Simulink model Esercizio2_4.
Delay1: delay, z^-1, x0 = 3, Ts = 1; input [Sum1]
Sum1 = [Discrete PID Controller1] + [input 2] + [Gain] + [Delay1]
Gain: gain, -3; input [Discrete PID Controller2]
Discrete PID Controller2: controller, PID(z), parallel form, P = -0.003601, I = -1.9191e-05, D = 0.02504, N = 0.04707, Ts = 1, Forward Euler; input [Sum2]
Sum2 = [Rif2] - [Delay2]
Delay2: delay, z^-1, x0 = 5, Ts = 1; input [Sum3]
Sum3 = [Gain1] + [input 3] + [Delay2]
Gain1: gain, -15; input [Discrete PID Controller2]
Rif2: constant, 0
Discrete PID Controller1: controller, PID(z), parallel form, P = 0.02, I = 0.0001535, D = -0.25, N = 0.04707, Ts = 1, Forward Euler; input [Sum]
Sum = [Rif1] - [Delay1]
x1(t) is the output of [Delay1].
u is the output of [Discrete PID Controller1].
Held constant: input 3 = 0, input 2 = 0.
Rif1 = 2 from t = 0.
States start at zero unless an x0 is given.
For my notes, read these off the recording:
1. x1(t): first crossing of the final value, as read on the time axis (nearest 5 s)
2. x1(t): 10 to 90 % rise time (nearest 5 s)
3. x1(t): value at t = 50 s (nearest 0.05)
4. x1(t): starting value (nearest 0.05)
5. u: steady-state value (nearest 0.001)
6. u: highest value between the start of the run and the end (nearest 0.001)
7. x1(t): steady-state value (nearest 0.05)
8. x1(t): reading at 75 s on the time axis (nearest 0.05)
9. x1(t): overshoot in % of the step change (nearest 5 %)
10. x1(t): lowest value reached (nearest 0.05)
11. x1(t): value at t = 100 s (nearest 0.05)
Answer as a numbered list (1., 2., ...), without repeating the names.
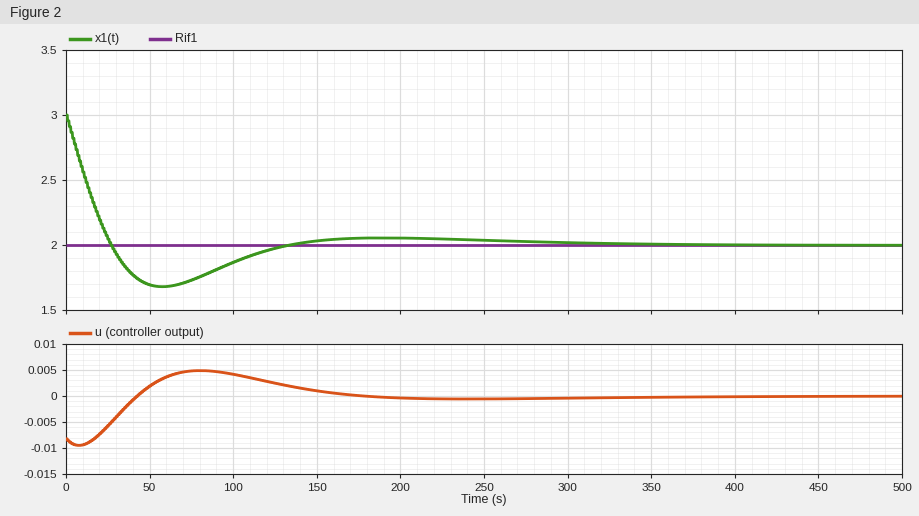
1. 25 s
2. 20 s
3. 1.70
4. 3.00
5. 0.000
6. 0.005
7. 2.00
8. 1.75
9. 30 %
10. 1.70
11. 1.85
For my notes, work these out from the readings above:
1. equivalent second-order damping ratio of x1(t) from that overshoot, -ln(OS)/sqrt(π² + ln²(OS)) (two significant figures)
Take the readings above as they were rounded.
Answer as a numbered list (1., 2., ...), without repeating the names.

1. 0.36
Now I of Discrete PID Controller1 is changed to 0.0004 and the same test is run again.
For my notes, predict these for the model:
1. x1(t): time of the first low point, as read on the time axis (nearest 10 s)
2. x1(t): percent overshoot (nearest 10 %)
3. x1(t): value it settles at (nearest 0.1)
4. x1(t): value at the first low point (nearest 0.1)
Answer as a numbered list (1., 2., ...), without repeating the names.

1. 60 s
2. 40 %
3. 2.0
4. 1.6
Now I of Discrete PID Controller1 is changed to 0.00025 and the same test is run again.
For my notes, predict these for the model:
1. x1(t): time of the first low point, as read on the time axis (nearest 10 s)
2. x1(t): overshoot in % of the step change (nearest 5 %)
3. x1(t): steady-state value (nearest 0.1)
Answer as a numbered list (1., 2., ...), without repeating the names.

1. 60 s
2. 35 %
3. 2.0
